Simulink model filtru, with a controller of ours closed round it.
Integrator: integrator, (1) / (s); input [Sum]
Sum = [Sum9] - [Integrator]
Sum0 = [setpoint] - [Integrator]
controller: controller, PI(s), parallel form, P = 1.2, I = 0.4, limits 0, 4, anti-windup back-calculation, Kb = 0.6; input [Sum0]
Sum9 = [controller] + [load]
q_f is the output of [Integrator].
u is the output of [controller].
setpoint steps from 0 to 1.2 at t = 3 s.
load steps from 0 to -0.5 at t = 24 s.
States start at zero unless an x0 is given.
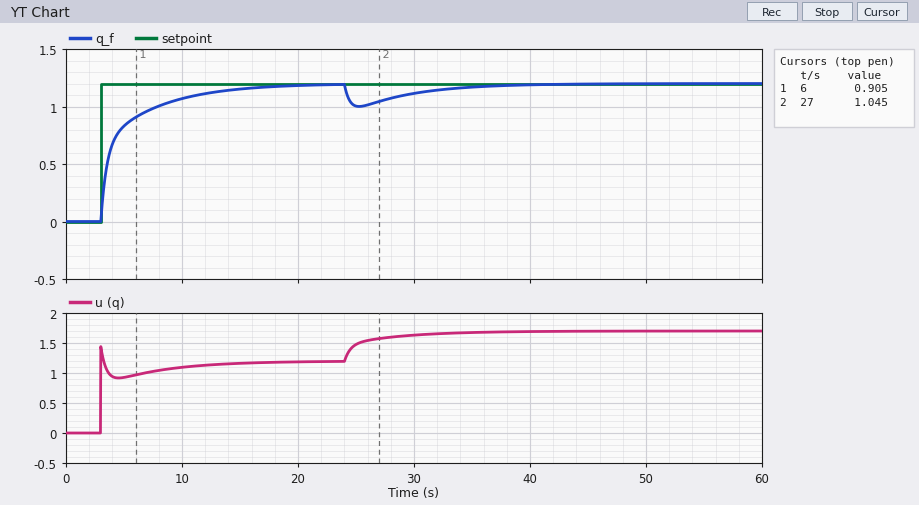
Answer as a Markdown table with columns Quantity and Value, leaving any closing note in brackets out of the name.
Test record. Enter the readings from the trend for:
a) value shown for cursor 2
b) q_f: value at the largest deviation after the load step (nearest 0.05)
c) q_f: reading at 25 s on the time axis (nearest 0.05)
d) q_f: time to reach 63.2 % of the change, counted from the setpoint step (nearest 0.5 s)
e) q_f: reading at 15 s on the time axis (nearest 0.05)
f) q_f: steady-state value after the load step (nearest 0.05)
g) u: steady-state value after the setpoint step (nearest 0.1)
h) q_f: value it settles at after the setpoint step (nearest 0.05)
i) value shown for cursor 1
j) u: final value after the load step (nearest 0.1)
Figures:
| Quantity | Value |
|---|---|
| value shown for cursor 2 | 1.045 |
| q_f: value at the largest deviation after the load step | 1.00 |
| q_f: reading at 25 s on the time axis | 1.00 |
| q_f: time to reach 63.2 % of the change, counted from the setpoint step | 1.5 s |
| q_f: reading at 15 s on the time axis | 1.15 |
| q_f: steady-state value after the load step | 1.20 |
| u: steady-state value after the setpoint step | 1.2 |
| q_f: value it settles at after the setpoint step | 1.20 |
| value shown for cursor 1 | 0.905 |
| u: final value after the load step | 1.7 |
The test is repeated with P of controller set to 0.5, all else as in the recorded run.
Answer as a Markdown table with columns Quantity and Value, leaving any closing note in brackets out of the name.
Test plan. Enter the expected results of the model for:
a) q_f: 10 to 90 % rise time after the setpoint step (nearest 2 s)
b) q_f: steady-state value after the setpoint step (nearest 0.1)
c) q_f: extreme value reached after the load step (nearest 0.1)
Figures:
| Quantity | Value |
|---|---|
| q_f: 10 to 90 % rise time after the setpoint step | 6 s |
| q_f: steady-state value after the setpoint step | 1.2 |
| q_f: extreme value reached after the load step | 0.9 |
